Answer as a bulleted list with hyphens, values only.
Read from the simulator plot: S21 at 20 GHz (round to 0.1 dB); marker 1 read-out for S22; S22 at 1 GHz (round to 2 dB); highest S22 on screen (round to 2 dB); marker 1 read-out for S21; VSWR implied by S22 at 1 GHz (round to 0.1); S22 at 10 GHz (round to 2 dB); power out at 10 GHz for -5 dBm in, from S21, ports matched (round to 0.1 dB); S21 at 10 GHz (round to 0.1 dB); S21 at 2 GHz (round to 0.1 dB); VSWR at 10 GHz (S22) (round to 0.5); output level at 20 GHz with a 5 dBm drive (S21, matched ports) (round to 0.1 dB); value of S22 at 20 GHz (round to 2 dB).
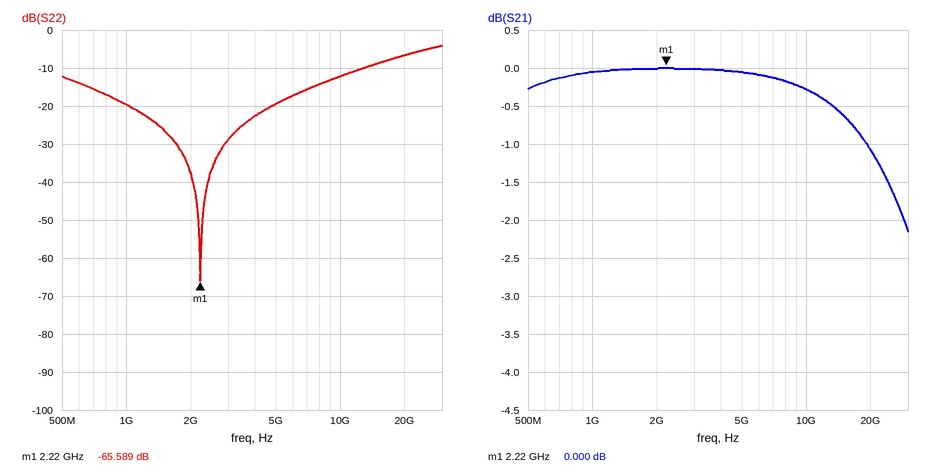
- -1.1 dB
- -65.589 dB
- -20 dB
- -4 dB
- 0.000 dB
- 1.2
- -12 dB
- -5.3 dBm
- -0.3 dB
- 0.0 dB
- 1.5
- 3.9 dBm
- -6 dB
